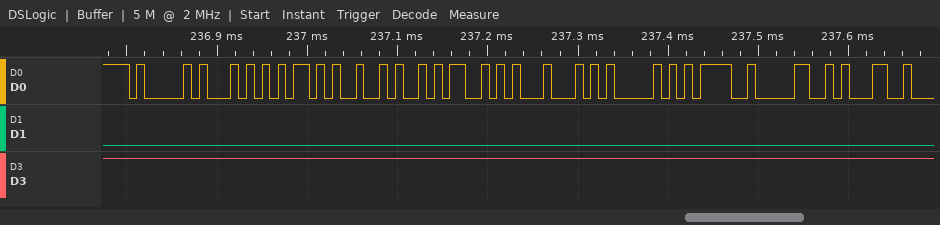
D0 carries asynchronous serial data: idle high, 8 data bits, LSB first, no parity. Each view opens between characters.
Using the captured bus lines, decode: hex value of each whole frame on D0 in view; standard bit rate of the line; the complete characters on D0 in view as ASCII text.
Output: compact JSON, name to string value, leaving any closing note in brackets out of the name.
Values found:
{"hex value of each whole frame on D0 in view": "41, 54, 2B, 4A, 53, 44, 41, 3D, 30, 31", "standard bit rate of the line": "115200 baud", "the complete characters on D0 in view as ASCII text": "\"AT+JSDA=01\""}
